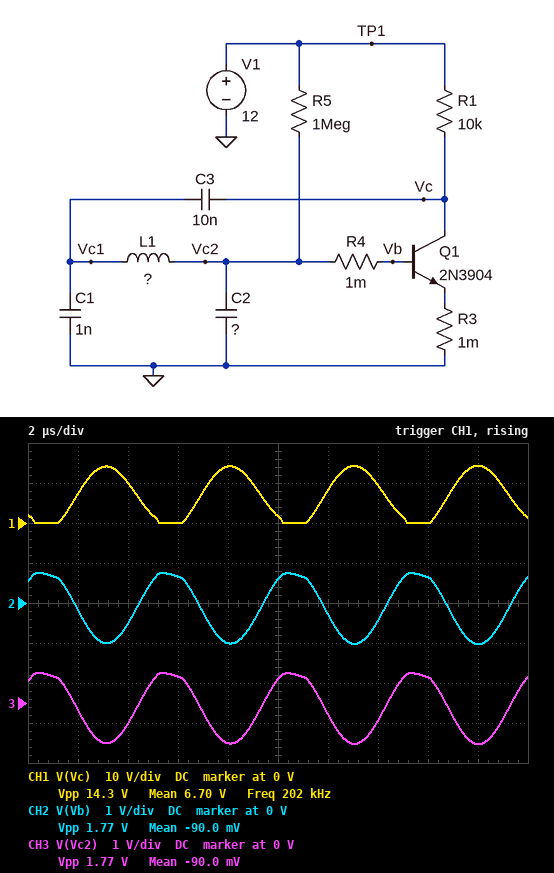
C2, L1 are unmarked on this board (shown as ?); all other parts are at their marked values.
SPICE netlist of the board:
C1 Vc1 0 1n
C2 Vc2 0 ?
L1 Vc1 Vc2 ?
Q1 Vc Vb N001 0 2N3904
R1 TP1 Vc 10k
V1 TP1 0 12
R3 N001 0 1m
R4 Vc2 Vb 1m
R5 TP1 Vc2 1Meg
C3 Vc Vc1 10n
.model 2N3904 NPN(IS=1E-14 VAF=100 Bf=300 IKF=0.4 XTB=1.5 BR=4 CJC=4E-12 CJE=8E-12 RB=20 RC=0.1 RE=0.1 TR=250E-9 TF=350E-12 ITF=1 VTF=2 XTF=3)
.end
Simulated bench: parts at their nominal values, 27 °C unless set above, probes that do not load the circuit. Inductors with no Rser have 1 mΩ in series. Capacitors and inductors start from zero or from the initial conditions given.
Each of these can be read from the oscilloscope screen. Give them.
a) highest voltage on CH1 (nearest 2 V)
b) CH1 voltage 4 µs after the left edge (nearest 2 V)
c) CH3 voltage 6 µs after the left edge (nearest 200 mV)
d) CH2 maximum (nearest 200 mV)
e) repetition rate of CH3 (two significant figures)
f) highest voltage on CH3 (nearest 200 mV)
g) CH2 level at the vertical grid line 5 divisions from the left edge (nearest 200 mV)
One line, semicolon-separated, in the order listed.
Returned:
14 V; 10 V; 600 mV; 800 mV; 200 kHz; 800 mV; 600 mV
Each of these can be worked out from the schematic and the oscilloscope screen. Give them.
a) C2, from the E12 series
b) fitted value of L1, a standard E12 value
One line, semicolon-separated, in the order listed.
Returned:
8.2 nF; 680 µH
